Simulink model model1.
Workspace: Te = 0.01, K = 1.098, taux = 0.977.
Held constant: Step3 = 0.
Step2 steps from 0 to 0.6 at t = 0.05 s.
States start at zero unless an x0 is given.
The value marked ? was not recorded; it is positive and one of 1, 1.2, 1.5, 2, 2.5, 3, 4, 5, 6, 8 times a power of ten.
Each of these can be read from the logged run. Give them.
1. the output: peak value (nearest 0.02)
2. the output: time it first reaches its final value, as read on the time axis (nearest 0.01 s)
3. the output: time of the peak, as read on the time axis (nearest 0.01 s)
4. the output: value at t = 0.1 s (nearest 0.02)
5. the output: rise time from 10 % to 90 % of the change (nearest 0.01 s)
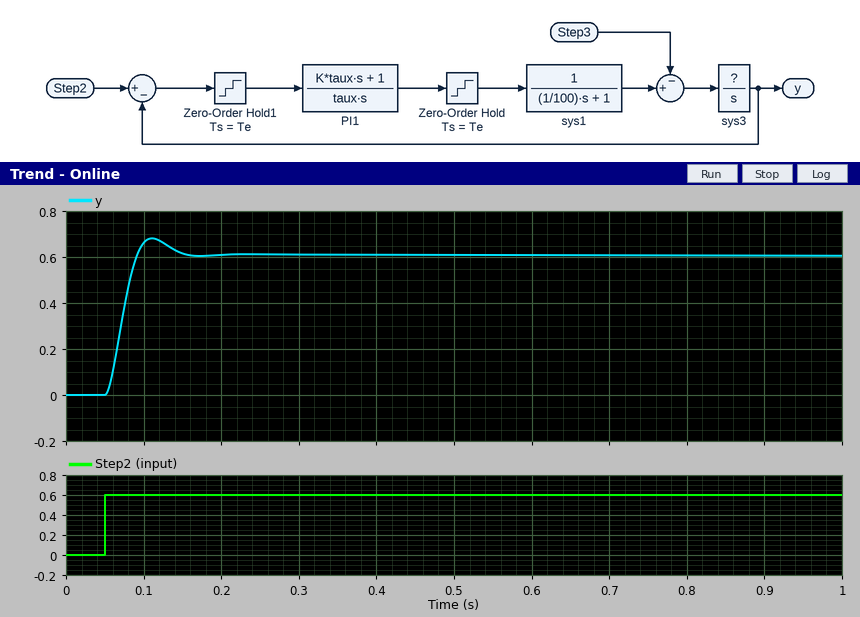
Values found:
0.68
0.09 s
0.11 s
0.66
0.03 s
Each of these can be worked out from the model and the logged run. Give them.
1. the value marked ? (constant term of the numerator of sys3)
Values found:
40
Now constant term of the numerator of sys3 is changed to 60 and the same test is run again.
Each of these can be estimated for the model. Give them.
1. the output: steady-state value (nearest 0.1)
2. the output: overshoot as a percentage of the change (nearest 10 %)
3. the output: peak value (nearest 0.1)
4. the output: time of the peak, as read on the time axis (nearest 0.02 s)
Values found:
0.6
30 %
0.8
0.10 s
